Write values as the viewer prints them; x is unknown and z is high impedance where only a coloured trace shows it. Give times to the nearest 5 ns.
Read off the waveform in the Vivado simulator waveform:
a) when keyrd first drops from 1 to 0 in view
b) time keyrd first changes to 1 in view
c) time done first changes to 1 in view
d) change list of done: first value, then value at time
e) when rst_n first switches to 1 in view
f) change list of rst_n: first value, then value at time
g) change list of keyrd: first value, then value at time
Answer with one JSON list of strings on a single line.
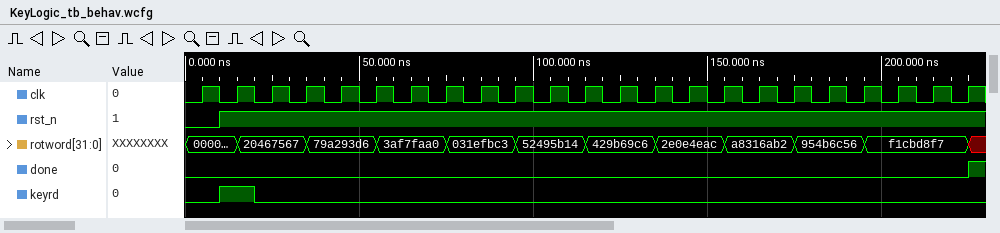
["20 ns", "10 ns", "225 ns", "0, 1 at 225 ns", "10 ns", "0, 1 at 10 ns", "0, 1 at 10 ns, 0 at 20 ns"]
